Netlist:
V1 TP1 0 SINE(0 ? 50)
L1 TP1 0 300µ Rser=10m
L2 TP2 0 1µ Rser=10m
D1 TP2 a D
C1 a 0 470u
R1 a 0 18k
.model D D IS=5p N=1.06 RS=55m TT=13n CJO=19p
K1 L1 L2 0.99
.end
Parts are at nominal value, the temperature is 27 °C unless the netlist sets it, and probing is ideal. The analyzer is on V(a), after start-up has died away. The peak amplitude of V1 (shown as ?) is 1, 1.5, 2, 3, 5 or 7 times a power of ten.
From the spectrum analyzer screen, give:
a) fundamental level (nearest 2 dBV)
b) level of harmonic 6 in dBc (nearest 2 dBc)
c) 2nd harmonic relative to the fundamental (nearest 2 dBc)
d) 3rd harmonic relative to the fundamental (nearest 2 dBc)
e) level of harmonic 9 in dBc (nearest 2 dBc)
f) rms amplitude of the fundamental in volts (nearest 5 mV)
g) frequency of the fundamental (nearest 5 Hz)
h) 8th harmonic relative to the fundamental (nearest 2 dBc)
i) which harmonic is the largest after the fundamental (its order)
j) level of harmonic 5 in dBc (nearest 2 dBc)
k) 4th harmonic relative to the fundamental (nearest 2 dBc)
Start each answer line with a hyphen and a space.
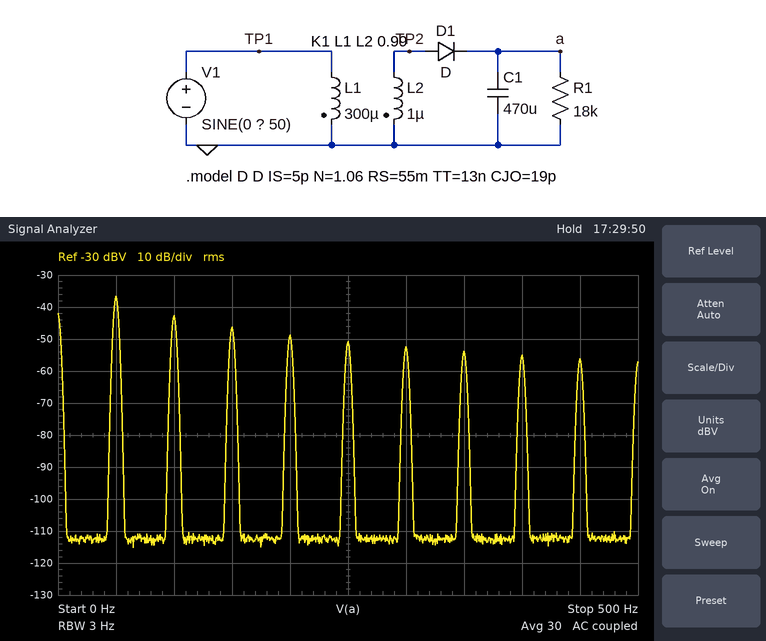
- -36 dBV
- -16 dBc
- -6 dBc
- -10 dBc
- -20 dBc
- 15 mV
- 50 Hz
- -18 dBc
- 2
- -14 dBc
- -12 dBc
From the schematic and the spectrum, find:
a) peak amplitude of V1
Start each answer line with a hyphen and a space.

- 500 V
